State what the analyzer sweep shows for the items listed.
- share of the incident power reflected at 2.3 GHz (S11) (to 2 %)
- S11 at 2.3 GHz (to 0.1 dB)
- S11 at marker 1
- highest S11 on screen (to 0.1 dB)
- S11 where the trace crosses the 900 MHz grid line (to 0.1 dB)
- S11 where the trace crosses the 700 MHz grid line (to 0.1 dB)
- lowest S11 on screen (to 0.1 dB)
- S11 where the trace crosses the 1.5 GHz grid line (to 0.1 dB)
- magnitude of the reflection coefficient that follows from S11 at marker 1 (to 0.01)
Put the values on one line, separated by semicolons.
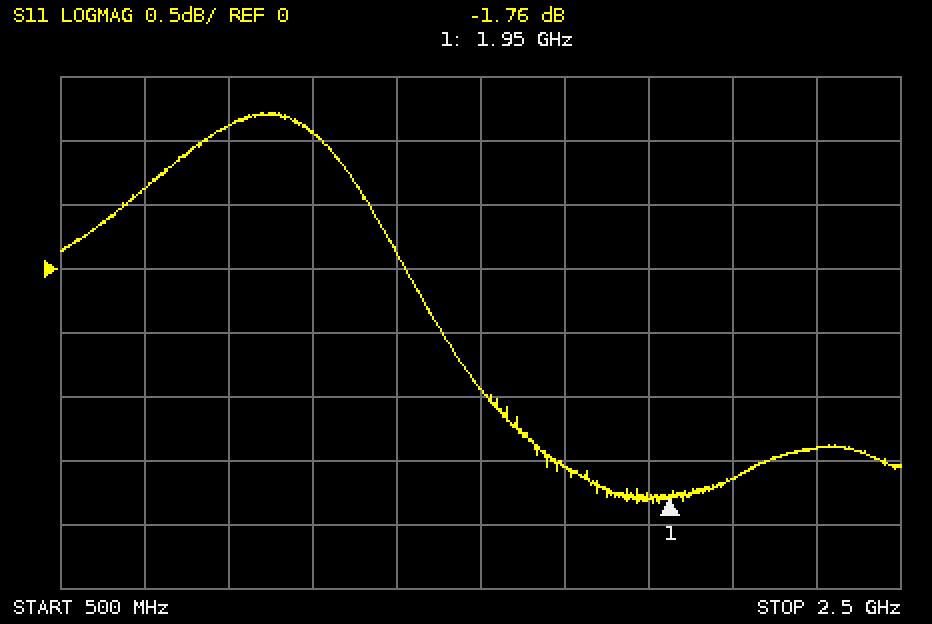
72 %; -1.4 dB; -1.76 dB; 1.2 dB; 1.1 dB; 0.6 dB; -1.8 dB; -0.9 dB; 0.82
